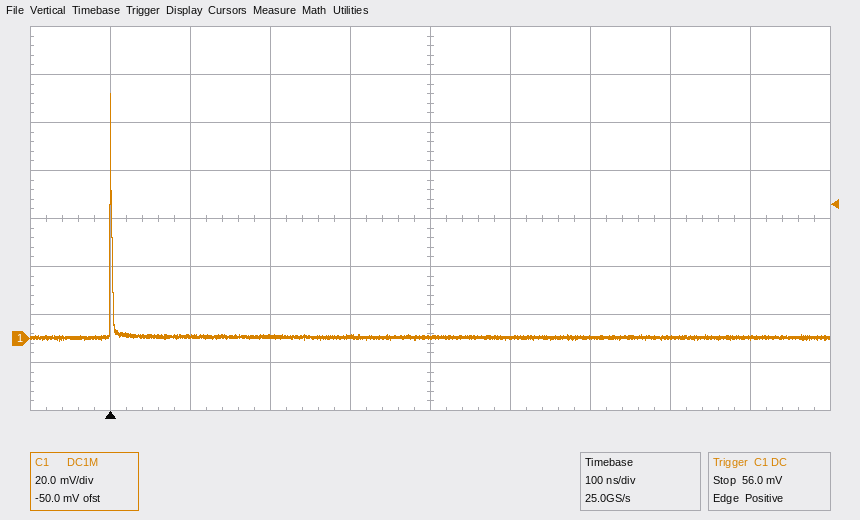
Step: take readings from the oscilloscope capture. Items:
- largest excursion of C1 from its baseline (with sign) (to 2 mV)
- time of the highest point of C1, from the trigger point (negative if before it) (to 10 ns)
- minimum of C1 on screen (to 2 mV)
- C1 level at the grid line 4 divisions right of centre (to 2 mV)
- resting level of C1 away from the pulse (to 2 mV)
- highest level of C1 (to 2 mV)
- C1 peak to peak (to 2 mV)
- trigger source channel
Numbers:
+102 mV
0 ns
-2 mV
0 mV
0 mV
102 mV
104 mV
C1
